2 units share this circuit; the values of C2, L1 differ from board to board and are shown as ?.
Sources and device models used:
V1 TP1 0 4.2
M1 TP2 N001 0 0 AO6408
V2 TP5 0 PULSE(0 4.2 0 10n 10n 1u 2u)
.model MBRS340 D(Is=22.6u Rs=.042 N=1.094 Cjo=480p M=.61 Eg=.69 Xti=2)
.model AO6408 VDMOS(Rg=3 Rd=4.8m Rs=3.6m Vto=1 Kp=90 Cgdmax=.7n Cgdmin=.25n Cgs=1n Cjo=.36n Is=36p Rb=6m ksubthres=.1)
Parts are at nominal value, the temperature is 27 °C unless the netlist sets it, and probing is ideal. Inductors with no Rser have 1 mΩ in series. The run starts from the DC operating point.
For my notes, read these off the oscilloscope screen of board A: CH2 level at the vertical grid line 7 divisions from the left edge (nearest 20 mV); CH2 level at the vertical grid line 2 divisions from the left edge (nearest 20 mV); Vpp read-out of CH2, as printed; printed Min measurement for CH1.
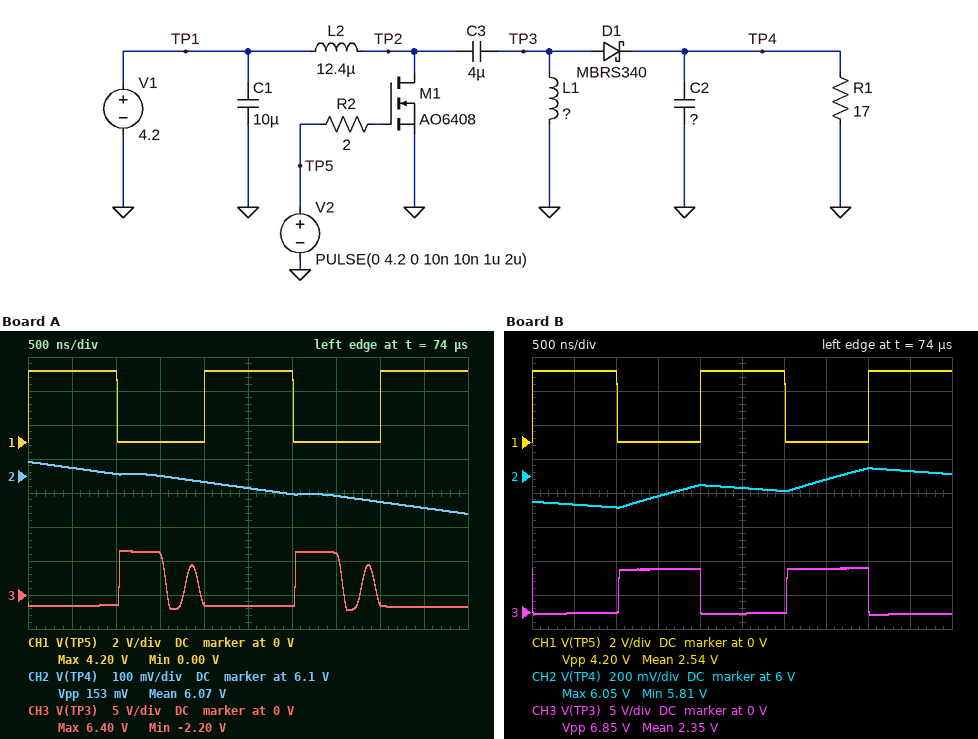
6.04 V
6.10 V
153 mV
0.00 V
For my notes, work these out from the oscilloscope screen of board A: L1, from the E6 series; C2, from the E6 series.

6.8 µH
10 µF
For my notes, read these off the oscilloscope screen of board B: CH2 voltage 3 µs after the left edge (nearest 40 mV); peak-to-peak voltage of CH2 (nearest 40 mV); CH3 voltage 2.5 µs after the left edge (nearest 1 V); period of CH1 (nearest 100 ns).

5.92 V
240 mV
0 V
2.0 µs
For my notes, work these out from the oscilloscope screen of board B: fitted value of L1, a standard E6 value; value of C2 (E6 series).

47 µH
10 µF
